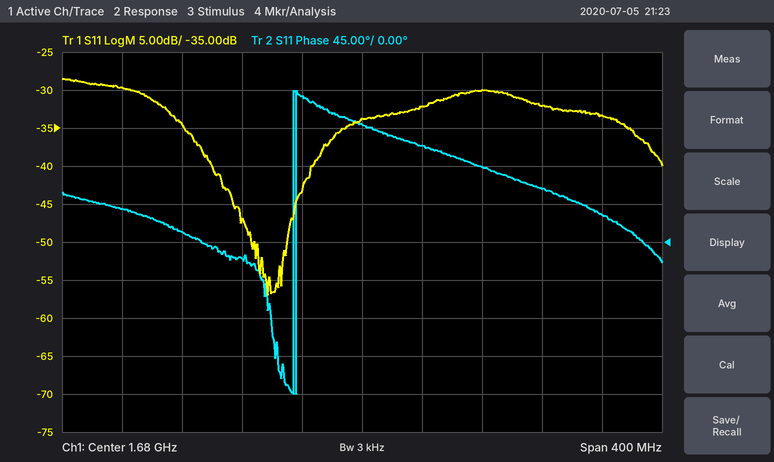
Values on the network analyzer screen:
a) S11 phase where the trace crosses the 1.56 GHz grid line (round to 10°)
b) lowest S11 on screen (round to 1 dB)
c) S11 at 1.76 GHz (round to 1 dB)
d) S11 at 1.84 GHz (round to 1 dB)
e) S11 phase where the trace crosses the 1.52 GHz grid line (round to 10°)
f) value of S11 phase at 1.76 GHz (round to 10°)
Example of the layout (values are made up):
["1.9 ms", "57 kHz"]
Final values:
["10°", "-57 dB", "-30 dB", "-33 dB", "40°", "90°"]
